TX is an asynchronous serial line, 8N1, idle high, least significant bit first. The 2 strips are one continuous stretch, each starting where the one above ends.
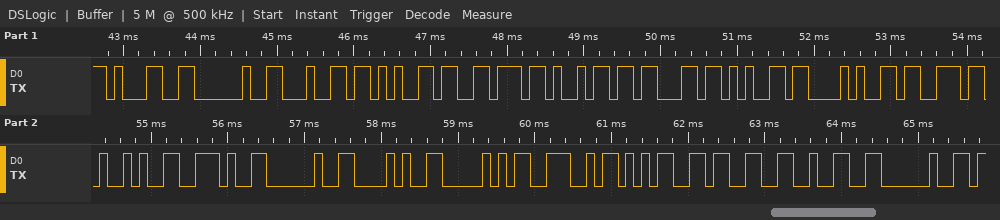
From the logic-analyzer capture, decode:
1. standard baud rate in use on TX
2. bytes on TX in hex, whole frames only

9600 baud
0x31 0x20 0x64 0x65 0x76 0x69 0x63 0x65 0x28 0x73 0x29 0x2E 0x20 0x28 0x50 0x4E 0x35 0x33 0x32 0x20
